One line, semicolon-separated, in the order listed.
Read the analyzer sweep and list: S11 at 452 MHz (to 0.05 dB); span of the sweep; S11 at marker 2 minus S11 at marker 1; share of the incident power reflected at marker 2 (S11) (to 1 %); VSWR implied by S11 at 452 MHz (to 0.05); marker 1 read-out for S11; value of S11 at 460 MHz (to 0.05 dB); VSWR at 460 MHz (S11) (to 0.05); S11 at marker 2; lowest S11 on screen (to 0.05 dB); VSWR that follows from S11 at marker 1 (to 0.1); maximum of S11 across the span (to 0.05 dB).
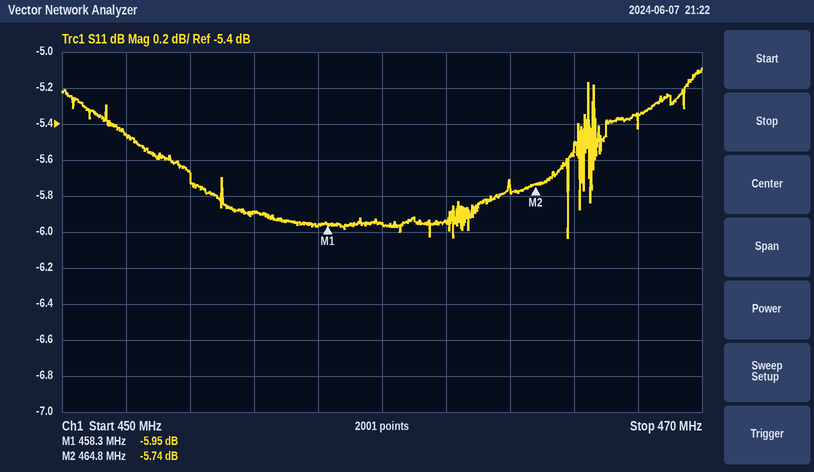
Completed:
-5.45 dB; 20 MHz; 0.21 dB; 27 %; 3.30; -5.95 dB; -5.95 dB; 3.05; -5.74 dB; -6.05 dB; 3.0; -5.10 dB
